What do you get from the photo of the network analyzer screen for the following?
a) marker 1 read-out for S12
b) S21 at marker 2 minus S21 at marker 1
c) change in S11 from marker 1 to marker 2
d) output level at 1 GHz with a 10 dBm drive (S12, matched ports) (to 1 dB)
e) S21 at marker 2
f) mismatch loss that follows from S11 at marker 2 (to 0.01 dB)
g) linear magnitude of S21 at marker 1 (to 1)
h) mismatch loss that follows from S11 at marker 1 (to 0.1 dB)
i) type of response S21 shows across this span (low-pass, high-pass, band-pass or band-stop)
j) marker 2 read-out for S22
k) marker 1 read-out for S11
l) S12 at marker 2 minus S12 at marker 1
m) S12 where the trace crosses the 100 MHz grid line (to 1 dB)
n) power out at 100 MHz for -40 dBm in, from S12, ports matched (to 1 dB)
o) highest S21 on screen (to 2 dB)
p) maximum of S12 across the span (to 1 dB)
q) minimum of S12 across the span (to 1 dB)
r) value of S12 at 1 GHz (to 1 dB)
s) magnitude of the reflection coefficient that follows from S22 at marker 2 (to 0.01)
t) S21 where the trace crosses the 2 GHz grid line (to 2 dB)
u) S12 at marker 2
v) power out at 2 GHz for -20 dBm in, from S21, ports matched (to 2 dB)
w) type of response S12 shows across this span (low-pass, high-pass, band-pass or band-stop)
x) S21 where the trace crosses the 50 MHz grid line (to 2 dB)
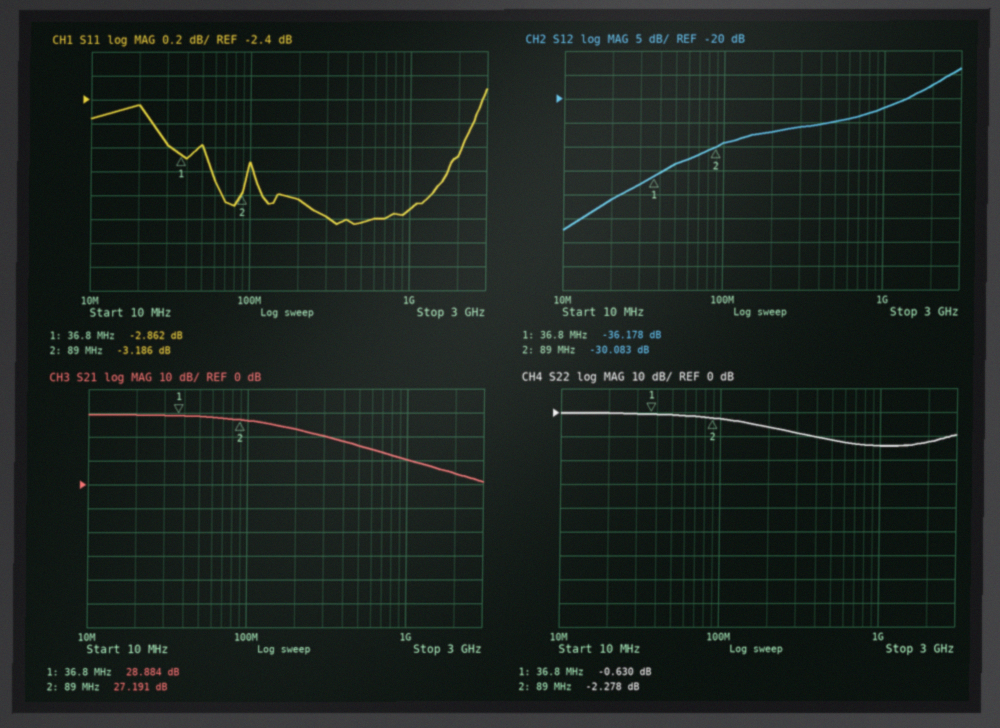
-36.178 dB
-1.693 dB
-0.324 dB
-12 dBm
27.191 dB
2.84 dB
28
3.2 dB
low-pass
-2.278 dB
-2.862 dB
6.095 dB
-29 dB
-69 dBm
30 dB
-14 dB
-47 dB
-22 dB
0.77
4 dB
-30.083 dB
-16 dBm
high-pass
28 dB
